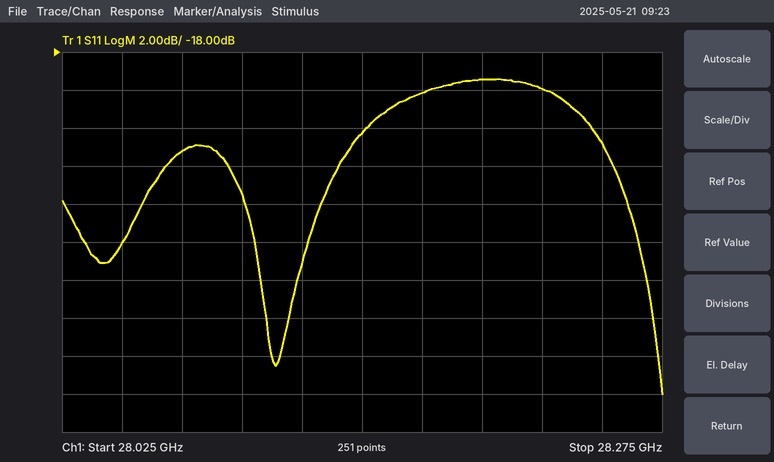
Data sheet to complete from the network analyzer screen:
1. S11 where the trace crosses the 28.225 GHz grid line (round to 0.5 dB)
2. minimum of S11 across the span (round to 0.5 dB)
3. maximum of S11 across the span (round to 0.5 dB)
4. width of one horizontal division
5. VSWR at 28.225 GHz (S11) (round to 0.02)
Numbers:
-20.0 dB
-36.0 dB
-19.5 dB
25 MHz
1.22
